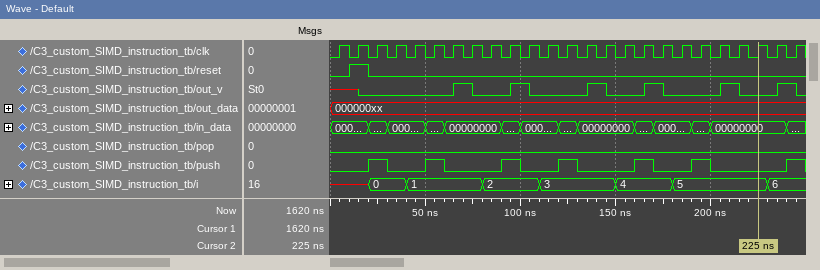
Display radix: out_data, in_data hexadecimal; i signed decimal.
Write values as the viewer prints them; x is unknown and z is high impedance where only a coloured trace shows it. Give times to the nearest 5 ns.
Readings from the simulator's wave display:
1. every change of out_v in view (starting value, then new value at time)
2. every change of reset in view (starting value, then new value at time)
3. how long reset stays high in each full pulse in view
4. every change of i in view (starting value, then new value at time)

x, 0 at 15 ns, 1 at 65 ns, 0 at 75 ns, 1 at 95 ns, 0 at 105 ns, 1 at 135 ns, 0 at 145 ns, 1 at 165 ns, 0 at 175 ns, 1 at 205 ns, 0 at 215 ns, 1 at 235 ns, 0 at 245 ns
0, 1 at 10 ns, 0 at 20 ns
10 ns
x, 0 at 20 ns, 1 at 40 ns, 2 at 80 ns, 3 at 110 ns, 4 at 150 ns, 5 at 180 ns, 6 at 230 ns
